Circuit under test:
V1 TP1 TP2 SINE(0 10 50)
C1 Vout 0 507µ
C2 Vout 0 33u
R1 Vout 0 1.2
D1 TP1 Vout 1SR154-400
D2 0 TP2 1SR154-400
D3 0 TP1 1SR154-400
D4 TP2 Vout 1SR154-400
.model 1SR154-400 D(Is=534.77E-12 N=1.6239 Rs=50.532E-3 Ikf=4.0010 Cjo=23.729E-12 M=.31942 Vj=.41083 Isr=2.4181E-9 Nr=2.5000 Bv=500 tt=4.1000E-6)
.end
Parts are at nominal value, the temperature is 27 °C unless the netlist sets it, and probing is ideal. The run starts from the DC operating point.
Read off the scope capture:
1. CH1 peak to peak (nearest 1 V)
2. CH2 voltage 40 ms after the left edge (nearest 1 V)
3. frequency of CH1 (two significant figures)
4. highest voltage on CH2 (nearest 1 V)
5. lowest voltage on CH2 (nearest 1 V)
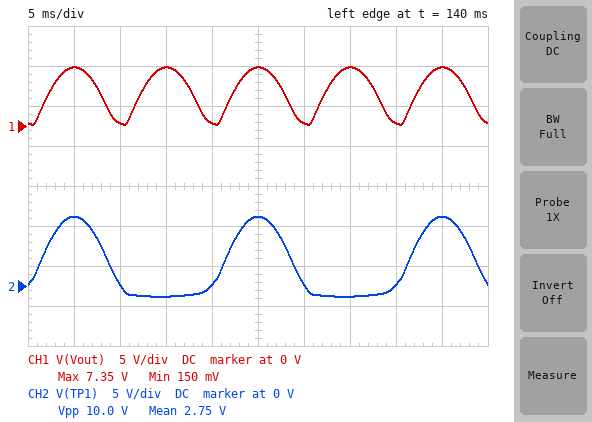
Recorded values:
7 V
0 V
100 Hz
9 V
-1 V
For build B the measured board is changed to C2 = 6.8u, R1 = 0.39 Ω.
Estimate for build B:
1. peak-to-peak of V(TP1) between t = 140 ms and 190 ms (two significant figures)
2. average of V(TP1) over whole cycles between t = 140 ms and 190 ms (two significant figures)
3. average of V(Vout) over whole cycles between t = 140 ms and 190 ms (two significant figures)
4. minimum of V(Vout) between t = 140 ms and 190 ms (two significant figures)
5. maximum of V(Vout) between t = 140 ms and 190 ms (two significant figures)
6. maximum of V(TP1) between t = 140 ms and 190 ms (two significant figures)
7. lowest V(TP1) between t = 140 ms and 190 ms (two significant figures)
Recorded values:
10 V
1.8 V
3.5 V
2.0 mV
6.2 V
8.1 V
-1.9 V
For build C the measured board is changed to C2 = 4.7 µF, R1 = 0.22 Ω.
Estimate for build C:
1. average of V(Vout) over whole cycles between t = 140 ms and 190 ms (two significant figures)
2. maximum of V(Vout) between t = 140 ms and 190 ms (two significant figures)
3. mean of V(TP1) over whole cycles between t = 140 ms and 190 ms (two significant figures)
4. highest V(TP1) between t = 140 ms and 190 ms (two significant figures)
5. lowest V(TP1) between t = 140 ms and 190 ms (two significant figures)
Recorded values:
3.0 V
5.3 V
1.5 V
7.7 V
-2.3 V
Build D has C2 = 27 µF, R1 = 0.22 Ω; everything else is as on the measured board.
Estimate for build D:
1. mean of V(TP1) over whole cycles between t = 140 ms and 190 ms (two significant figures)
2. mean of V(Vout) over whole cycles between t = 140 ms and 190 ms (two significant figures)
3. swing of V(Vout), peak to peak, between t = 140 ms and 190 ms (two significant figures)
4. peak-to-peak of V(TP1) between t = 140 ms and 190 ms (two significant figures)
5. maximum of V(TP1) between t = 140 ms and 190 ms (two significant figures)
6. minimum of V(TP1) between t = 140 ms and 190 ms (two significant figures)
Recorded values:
1.5 V
3.0 V
5.3 V
10 V
7.7 V
-2.3 V
